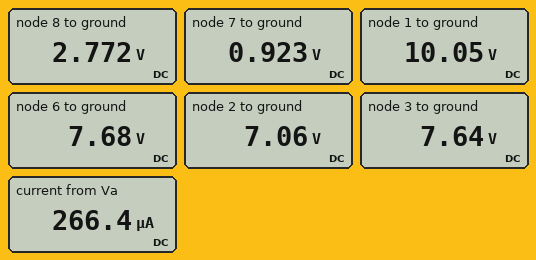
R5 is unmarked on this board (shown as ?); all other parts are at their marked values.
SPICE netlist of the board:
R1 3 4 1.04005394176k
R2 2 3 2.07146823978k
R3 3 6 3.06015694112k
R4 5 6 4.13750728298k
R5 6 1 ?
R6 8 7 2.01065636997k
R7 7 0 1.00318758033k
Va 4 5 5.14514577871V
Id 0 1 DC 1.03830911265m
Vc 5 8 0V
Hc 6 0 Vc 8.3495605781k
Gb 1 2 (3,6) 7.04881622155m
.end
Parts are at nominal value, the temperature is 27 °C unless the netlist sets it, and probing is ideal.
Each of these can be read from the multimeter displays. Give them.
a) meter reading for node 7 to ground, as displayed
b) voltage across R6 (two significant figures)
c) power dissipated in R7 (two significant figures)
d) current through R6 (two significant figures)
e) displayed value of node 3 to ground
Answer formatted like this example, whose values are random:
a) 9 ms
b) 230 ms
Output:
a) 0.923 V
b) 1.8 V
c) 850 µW
d) 920 µA
e) 7.64 V
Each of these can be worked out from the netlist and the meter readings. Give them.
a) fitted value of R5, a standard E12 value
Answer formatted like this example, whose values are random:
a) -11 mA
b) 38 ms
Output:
a) 1.8 kΩ
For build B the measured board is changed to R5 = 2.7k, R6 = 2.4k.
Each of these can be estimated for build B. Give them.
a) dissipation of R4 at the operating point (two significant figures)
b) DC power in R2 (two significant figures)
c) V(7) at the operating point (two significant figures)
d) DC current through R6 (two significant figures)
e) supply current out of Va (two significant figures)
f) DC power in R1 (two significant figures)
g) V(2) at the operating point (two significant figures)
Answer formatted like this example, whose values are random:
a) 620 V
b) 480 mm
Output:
a) 6.0 mW
b) 88 µW
c) 1.0 V
d) 1.0 mA
e) 200 µA
f) 40 µW
g) 7.9 V
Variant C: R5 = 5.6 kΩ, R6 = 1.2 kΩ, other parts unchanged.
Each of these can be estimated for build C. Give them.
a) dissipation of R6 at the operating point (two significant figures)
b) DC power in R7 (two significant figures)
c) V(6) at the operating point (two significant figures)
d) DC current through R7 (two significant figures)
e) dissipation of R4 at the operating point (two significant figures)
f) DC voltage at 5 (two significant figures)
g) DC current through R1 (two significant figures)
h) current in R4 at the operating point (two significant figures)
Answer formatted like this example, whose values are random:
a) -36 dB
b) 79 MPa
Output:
a) 730 µW
b) 610 µW
c) 6.5 V
d) 780 µA
e) 5.6 mW
f) 1.7 V
g) 380 µA
h) 1.2 mA
